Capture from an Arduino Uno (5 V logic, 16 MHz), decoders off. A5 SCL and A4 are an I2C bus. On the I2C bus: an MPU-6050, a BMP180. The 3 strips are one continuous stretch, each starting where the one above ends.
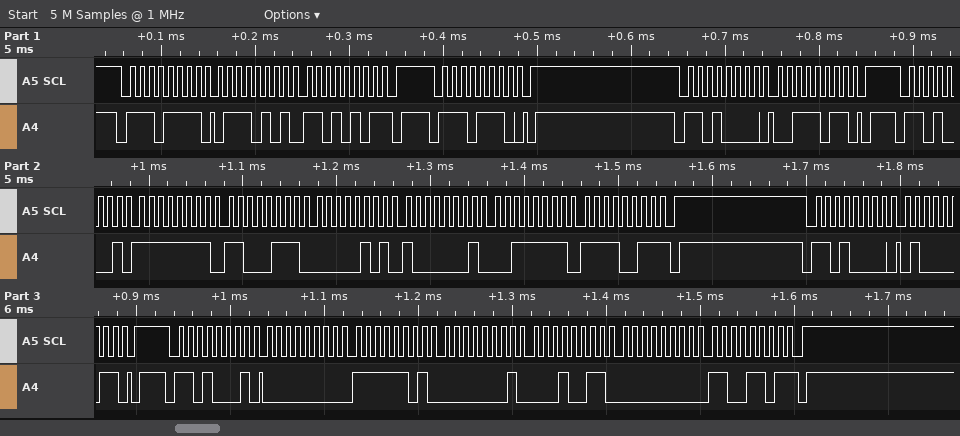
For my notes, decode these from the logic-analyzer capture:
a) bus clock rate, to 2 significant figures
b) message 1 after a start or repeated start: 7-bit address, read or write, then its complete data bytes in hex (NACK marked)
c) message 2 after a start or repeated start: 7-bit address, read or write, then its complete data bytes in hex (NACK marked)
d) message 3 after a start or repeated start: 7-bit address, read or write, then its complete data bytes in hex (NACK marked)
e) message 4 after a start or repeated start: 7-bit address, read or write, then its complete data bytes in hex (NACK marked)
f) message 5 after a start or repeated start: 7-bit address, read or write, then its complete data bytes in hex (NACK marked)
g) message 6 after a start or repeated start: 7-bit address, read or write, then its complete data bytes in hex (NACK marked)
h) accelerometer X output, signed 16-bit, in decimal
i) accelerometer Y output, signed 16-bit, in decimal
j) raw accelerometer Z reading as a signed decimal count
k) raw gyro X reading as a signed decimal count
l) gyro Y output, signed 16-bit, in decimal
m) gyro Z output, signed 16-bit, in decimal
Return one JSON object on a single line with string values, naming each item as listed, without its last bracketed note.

{"bus clock rate, to 2 significant figures": "100 kHz", "message 1 after a start or repeated start: 7-bit address, read or write, then its complete data bytes in hex": "0x77 read: 75 D5 NACK", "message 2 after a start or repeated start: 7-bit address, read or write, then its complete data bytes in hex": "0x77 write", "message 3 after a start or repeated start: 7-bit address, read or write, then its complete data bytes in hex": "0x68 write: 3B", "message 4 after a start or repeated start: 7-bit address, read or write, then its complete data bytes in hex": "0x68 read: FF C7 05 81 3F F3 NACK", "message 5 after a start or repeated start: 7-bit address, read or write, then its complete data bytes in hex": "0x68 write: 43", "message 6 after a start or repeated start: 7-bit address, read or write, then its complete data bytes in hex": "0x68 read: 00 FD 01 13 00 CD NACK", "accelerometer X output, signed 16-bit, in decimal": "-57", "accelerometer Y output, signed 16-bit, in decimal": "1409", "raw accelerometer Z reading as a signed decimal count": "16371", "raw gyro X reading as a signed decimal count": "253", "gyro Y output, signed 16-bit, in decimal": "275", "gyro Z output, signed 16-bit, in decimal": "205"}
